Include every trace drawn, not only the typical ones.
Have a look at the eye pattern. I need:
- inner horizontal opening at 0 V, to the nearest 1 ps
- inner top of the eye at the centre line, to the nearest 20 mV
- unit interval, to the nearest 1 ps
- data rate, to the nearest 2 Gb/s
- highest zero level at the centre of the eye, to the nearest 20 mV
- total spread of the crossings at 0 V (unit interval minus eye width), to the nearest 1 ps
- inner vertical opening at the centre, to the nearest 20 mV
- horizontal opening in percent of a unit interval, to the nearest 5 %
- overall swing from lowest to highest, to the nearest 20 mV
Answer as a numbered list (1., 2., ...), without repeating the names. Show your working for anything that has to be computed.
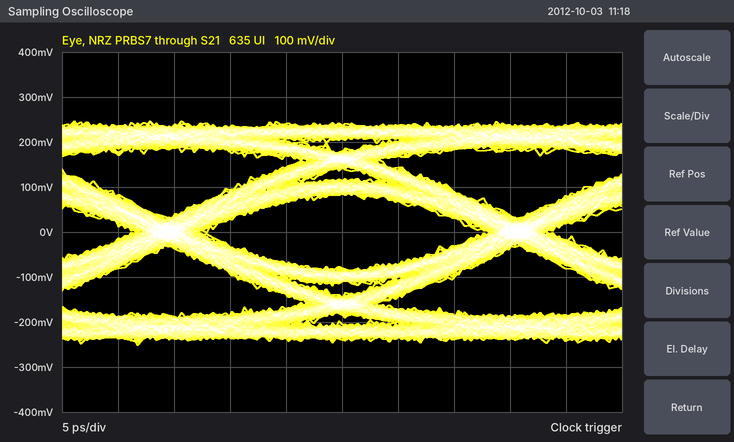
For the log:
1. 25 ps
2. 80 mV
3. 31 ps
4. 32 Gb/s
5. -80 mV
6. 6 ps
7. 160 mV
8. 25 ps / 31 ps ≈ 80.6 %, so 80 % to the nearest 5 %
9. 500 mV
